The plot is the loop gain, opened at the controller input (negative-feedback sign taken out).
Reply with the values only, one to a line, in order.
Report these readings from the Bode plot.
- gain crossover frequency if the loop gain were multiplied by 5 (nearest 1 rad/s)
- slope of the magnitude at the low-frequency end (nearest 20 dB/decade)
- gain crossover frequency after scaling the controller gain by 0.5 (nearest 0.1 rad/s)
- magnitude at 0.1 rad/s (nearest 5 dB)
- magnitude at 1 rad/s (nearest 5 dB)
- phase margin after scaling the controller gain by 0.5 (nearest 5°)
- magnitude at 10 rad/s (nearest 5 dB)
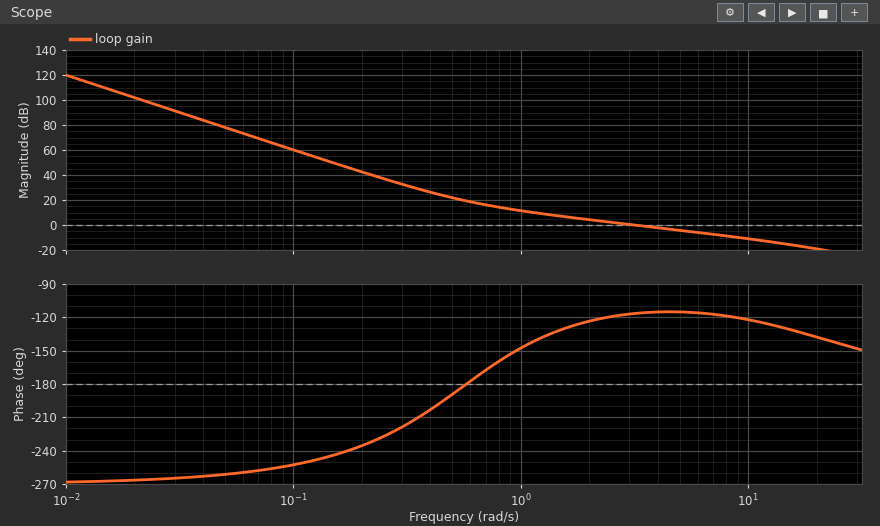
13 rad/s
-60 dB/decade
1.7 rad/s
60 dB
10 dB
50°
-10 dB
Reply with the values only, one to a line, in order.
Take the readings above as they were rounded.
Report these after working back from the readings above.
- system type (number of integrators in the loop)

3
